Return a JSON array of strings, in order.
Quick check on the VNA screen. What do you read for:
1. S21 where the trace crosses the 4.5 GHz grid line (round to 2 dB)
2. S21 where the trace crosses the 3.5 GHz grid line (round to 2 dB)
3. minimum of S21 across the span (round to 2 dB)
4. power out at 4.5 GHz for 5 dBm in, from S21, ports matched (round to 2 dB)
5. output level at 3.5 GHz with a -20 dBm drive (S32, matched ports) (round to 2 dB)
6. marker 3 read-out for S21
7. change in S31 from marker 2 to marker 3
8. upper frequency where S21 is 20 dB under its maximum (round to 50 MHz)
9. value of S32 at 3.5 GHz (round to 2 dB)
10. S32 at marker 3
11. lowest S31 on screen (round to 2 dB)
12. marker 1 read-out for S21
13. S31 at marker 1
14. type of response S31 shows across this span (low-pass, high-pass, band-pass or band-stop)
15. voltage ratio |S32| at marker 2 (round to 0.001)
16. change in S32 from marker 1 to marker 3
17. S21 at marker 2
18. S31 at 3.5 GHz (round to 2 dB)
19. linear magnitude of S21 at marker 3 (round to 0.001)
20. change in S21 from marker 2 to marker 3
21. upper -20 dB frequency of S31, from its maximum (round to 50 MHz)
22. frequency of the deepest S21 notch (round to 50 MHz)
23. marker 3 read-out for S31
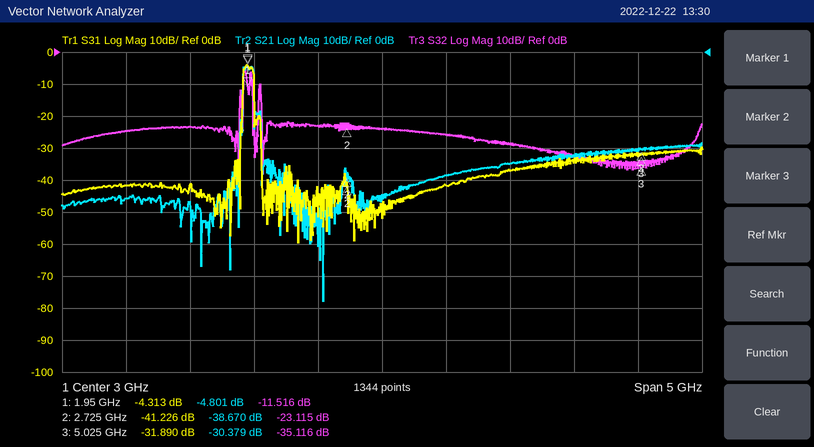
["-32 dB", "-38 dB", "-78 dB", "-28 dBm", "-46 dBm", "-30.379 dB", "9.336 dB", "2.05 GHz", "-26 dB", "-35.116 dB", "-60 dB", "-4.801 dB", "-4.313 dB", "band-pass", "0.070", "-23.600 dB", "-38.670 dB", "-42 dB", "0.030", "8.291 dB", "2.05 GHz", "2.55 GHz", "-31.890 dB"]
